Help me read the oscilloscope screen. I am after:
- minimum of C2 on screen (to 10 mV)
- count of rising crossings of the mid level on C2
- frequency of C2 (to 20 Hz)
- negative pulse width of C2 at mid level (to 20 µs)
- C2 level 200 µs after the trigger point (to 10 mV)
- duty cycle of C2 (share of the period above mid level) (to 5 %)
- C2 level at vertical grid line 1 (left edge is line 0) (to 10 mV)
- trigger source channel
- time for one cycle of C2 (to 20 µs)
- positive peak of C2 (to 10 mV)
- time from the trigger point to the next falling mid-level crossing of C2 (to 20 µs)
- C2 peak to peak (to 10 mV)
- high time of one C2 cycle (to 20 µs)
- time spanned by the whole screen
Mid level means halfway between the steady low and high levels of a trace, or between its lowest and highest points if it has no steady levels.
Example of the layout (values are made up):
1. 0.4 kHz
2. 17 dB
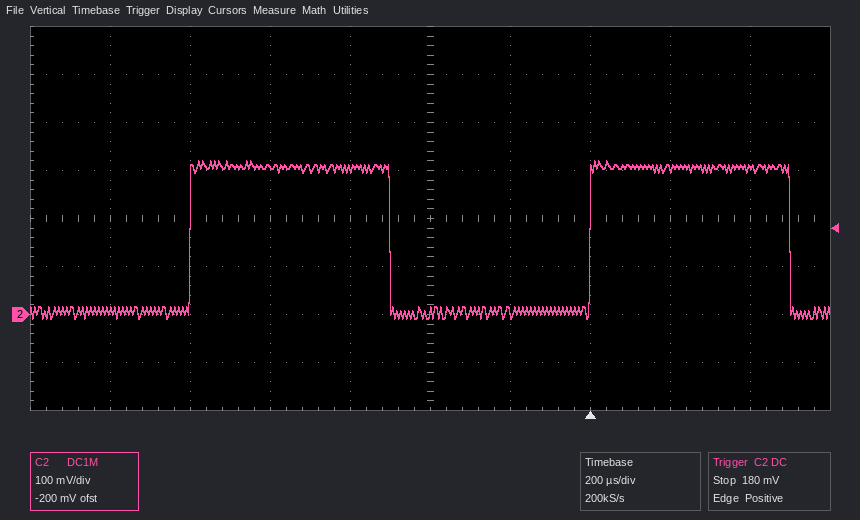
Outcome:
1. -10 mV
2. 2
3. 1.00 kHz
4. 500 µs
5. 300 mV
6. 50 %
7. 10 mV
8. C2
9. 1.00 ms
10. 320 mV
11. 500 µs
12. 330 mV
13. 500 µs
14. 2 ms
